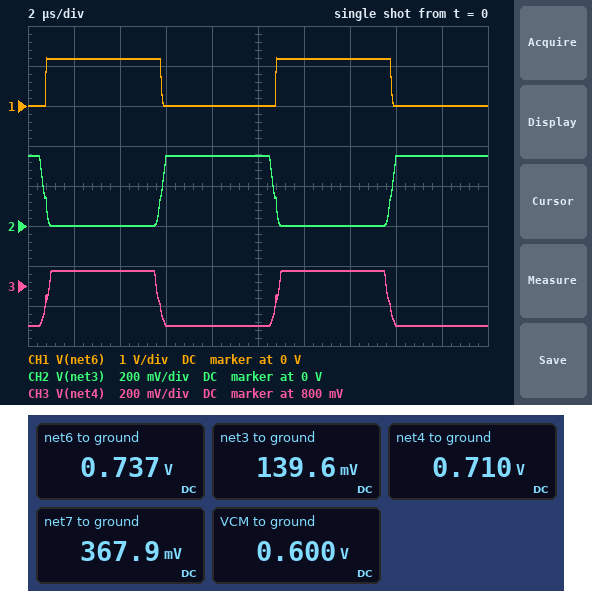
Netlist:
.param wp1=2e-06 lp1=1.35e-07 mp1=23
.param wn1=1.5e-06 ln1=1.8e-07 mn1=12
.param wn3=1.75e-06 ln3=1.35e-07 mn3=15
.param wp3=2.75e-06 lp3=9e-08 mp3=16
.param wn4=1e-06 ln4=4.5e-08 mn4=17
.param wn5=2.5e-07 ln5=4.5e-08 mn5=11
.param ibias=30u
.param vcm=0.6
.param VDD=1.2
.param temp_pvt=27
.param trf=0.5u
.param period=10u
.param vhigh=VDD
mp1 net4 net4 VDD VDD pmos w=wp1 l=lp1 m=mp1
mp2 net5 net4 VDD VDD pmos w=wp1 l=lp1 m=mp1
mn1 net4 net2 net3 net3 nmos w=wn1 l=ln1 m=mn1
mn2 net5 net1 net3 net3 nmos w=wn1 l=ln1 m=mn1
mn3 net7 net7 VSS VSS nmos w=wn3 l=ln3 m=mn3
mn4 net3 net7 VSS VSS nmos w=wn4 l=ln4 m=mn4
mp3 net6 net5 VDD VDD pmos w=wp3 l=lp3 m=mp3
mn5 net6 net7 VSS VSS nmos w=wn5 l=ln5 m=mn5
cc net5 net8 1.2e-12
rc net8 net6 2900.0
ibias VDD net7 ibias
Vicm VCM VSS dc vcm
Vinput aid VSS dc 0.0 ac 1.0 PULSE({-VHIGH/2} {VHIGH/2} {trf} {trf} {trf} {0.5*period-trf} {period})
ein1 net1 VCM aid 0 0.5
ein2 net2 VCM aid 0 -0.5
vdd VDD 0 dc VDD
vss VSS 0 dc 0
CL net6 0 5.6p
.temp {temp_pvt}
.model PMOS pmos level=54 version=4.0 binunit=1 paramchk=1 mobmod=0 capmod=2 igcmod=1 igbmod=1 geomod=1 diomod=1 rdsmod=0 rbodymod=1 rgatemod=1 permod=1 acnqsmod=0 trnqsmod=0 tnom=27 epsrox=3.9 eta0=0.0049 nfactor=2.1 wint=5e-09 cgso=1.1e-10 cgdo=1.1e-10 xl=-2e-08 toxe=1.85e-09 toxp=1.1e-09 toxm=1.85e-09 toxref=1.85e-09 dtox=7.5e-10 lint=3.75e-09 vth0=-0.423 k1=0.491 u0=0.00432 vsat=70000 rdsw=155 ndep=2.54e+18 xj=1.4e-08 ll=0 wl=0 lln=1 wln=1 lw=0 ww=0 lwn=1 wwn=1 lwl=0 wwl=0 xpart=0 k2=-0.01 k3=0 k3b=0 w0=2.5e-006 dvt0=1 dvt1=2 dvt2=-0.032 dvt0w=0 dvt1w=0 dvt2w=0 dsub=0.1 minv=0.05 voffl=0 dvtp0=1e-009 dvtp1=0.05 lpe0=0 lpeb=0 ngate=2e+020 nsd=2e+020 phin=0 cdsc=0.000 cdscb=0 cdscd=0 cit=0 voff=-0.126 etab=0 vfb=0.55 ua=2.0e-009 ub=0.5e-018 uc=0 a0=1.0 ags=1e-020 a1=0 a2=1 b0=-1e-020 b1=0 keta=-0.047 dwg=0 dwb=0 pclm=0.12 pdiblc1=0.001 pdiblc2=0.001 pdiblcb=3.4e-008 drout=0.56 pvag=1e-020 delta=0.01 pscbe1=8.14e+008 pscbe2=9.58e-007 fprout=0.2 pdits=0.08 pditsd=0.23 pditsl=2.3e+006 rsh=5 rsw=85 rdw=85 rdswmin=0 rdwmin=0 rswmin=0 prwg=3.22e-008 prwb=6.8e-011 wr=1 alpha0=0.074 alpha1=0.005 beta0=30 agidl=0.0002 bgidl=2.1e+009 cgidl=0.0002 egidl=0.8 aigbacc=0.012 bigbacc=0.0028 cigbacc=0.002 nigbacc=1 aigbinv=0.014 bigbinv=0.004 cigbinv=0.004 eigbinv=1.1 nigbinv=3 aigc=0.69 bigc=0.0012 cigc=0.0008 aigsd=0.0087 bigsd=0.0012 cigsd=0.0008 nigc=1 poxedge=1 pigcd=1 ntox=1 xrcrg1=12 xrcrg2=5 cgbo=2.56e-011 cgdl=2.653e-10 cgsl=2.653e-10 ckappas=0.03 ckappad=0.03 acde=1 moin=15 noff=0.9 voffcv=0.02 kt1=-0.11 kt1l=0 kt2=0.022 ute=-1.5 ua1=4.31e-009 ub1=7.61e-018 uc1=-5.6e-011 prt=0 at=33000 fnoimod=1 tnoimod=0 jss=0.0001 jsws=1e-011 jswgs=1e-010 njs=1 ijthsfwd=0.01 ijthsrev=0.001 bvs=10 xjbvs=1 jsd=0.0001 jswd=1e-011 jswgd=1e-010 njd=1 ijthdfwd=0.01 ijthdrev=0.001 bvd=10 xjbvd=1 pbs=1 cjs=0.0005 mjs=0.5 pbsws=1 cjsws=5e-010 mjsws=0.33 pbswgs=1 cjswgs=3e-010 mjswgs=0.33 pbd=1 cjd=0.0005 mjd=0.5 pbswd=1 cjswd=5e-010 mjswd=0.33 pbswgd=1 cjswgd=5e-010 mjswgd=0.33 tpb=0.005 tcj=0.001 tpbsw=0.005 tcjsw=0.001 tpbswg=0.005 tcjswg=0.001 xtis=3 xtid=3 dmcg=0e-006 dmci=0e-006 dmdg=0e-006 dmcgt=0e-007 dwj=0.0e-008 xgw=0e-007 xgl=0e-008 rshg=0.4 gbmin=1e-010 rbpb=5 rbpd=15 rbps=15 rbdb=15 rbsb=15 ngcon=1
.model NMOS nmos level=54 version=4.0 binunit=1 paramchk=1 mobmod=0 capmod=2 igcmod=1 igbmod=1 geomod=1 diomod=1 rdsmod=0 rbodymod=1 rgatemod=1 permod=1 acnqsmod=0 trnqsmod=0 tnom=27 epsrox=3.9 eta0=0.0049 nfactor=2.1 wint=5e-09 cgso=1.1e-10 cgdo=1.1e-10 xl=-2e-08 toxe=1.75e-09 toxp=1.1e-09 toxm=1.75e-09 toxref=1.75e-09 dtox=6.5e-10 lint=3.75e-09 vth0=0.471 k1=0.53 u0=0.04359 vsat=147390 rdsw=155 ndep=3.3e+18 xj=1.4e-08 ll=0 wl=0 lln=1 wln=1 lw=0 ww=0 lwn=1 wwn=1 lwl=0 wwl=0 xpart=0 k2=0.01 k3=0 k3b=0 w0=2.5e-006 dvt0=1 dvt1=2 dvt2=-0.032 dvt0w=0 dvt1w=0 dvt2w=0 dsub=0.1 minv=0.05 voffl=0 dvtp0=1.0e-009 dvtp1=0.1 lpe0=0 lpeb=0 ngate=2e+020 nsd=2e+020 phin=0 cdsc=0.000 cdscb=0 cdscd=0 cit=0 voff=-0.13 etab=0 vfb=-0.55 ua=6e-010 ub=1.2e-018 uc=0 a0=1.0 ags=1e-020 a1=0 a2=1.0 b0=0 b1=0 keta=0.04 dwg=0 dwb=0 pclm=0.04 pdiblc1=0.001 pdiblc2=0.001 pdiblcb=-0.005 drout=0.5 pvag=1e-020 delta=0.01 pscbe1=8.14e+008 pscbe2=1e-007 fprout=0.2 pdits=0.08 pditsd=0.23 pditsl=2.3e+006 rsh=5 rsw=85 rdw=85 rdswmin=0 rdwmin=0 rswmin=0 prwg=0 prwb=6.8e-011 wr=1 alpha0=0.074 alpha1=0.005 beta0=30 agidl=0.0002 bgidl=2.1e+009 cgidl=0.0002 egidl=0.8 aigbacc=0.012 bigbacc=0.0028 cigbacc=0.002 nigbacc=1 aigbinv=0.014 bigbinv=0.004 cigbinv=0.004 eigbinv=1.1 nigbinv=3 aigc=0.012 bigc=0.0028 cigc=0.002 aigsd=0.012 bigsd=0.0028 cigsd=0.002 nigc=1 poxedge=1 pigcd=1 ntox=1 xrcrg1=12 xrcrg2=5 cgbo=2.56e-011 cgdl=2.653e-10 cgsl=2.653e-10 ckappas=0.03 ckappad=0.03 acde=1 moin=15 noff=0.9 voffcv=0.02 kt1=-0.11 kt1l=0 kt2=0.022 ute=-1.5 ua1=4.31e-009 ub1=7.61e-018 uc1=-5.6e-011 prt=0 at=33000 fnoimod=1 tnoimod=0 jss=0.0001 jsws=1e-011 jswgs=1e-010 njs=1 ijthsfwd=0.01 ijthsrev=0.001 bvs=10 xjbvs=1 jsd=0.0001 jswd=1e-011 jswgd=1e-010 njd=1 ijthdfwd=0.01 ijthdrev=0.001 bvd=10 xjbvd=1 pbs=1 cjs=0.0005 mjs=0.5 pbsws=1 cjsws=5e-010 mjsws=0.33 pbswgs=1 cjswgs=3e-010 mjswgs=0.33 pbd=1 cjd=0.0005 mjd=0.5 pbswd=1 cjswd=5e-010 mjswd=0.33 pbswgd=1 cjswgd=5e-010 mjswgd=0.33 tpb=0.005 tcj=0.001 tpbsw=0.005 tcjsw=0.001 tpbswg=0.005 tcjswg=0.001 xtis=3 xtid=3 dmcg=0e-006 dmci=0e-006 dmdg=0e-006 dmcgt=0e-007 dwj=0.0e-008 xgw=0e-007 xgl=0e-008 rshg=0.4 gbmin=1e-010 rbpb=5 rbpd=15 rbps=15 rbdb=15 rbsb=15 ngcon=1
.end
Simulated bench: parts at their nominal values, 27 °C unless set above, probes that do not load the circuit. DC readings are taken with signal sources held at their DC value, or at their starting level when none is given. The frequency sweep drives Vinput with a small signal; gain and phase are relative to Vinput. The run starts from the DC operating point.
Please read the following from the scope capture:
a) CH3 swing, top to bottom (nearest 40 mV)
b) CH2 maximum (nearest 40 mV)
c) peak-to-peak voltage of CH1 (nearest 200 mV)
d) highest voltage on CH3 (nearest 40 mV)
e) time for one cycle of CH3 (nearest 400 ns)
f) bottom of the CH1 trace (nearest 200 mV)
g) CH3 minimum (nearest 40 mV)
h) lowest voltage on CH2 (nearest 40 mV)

280 mV
360 mV
1.2 V
880 mV
10.0 µs
0 V
600 mV
0 V
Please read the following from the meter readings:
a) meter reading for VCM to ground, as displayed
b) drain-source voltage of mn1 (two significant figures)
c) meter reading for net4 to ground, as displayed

0.600 V
570 mV
0.710 V
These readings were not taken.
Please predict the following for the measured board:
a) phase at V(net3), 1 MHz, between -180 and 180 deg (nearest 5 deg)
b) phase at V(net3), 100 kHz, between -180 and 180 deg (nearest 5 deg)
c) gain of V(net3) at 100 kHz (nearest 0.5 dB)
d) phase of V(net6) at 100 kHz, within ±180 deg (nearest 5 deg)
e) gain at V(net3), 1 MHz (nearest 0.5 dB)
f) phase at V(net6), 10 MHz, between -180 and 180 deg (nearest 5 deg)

120 deg
165 deg
-16.5 dB
-15 deg
-24.5 dB
-85 deg
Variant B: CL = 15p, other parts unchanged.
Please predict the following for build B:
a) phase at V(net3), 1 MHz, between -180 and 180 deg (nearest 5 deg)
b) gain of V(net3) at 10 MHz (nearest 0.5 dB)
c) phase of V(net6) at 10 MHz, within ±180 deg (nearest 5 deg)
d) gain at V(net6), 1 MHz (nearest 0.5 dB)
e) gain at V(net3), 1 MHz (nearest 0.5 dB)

125 deg
-36.5 dB
-100 deg
43.0 dB
-25.0 dB
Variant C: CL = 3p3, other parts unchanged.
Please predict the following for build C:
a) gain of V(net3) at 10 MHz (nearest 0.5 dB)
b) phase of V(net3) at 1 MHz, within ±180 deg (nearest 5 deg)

-42.0 dB
115 deg
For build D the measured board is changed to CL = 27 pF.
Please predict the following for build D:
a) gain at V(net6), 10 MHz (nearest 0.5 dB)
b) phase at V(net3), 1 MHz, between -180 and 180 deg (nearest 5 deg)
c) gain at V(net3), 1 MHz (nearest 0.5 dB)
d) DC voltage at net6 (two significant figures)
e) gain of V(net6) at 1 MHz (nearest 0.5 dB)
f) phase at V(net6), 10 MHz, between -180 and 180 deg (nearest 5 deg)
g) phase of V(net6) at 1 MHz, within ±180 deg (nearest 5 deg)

22.0 dB
130 deg
-25.0 dB
740 mV
42.5 dB
-110 deg
-75 deg
